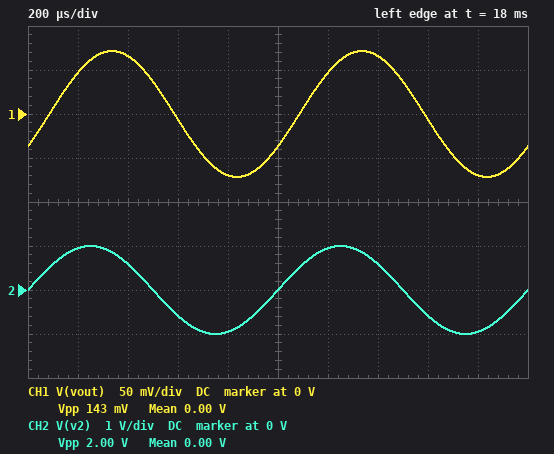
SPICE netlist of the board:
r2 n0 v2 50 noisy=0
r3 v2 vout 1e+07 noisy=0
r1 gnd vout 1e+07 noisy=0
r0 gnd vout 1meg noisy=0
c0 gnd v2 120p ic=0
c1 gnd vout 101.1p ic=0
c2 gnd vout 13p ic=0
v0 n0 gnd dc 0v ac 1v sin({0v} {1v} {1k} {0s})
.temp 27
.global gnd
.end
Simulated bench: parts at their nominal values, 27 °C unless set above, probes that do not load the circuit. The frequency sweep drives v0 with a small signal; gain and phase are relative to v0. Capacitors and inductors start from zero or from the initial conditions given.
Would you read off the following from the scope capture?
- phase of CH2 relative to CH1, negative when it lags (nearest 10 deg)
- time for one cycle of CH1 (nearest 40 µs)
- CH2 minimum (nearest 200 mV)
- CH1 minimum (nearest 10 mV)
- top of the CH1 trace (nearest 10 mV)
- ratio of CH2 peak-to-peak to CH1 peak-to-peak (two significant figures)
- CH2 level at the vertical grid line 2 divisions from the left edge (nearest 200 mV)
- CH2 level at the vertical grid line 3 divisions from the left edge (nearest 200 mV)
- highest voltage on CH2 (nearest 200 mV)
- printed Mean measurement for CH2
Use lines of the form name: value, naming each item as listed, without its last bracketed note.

phase of CH2 relative to CH1, negative when it lags: 30 deg
time for one cycle of CH1: 1.00 ms
CH2 minimum: -1.0 V
CH1 minimum: -70 mV
top of the CH1 trace: 70 mV
ratio of CH2 peak-to-peak to CH1 peak-to-peak: 14
CH2 level at the vertical grid line 2 divisions from the left edge: 600 mV
CH2 level at the vertical grid line 3 divisions from the left edge: -600 mV
highest voltage on CH2: 1.0 V
printed Mean measurement for CH2: 0.00 V
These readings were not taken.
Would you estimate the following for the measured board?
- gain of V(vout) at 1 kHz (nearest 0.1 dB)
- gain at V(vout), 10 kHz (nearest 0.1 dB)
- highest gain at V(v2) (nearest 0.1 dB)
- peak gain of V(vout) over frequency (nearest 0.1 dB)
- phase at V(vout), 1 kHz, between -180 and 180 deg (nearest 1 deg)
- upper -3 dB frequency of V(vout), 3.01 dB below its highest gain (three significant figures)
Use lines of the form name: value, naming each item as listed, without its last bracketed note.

gain of V(vout) at 1 kHz: -22.9 dB
gain at V(vout), 10 kHz: -37.2 dB
highest gain at V(v2): 0 dB
peak gain of V(vout) over frequency: -21.6 dB
phase at V(vout), 1 kHz, between -180 and 180 deg: -31 deg
upper -3 dB frequency of V(vout), 3.01 dB below its highest gain: 1.67 kHz
